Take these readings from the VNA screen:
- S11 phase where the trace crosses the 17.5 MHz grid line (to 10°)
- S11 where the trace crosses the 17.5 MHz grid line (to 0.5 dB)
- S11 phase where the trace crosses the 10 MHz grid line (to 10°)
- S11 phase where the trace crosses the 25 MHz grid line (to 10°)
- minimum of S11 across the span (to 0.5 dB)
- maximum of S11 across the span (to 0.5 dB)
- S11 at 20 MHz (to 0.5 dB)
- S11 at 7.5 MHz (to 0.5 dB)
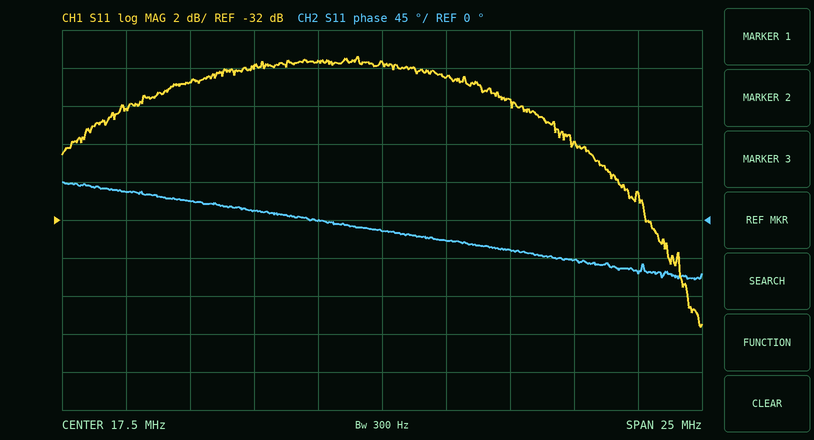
-10°
-23.5 dB
20°
-50°
-37.5 dB
-23.5 dB
-24.5 dB
-26.0 dB
